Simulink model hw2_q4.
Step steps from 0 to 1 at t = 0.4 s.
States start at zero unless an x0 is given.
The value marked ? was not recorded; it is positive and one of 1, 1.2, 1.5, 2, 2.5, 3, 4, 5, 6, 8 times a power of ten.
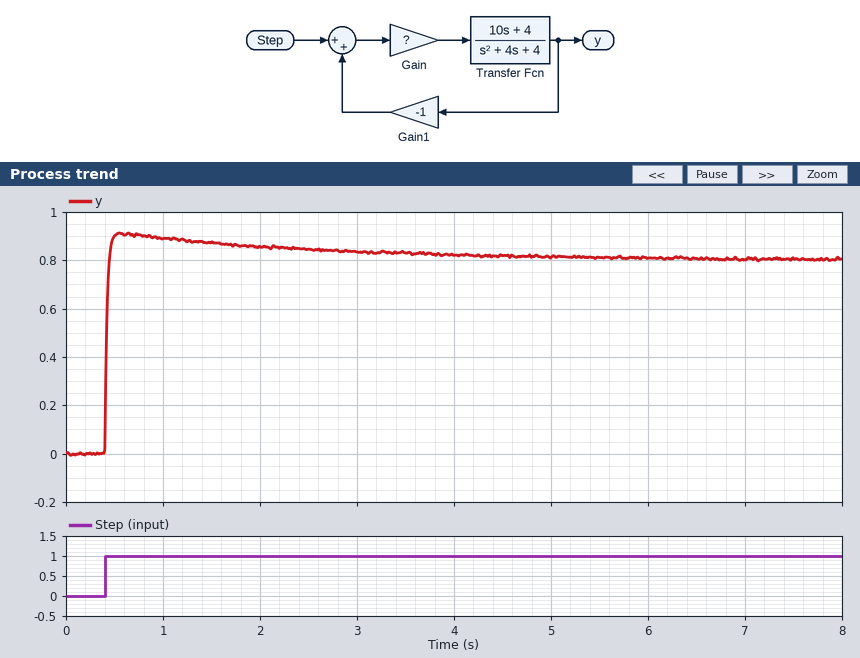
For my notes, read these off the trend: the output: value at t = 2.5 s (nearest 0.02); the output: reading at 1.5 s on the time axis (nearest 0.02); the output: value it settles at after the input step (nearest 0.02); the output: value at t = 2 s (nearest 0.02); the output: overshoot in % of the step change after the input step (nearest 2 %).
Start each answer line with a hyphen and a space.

- 0.84
- 0.88
- 0.80
- 0.86
- 14 %
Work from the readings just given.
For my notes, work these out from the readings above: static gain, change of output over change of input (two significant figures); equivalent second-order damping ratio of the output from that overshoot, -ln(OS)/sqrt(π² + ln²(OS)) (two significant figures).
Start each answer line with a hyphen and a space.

- 0.80
- 0.53
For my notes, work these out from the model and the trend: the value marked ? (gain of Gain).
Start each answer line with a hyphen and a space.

- 4
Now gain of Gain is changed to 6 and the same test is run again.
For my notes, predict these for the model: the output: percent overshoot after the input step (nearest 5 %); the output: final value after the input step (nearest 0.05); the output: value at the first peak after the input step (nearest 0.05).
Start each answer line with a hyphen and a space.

- 10 %
- 0.85
- 0.95
